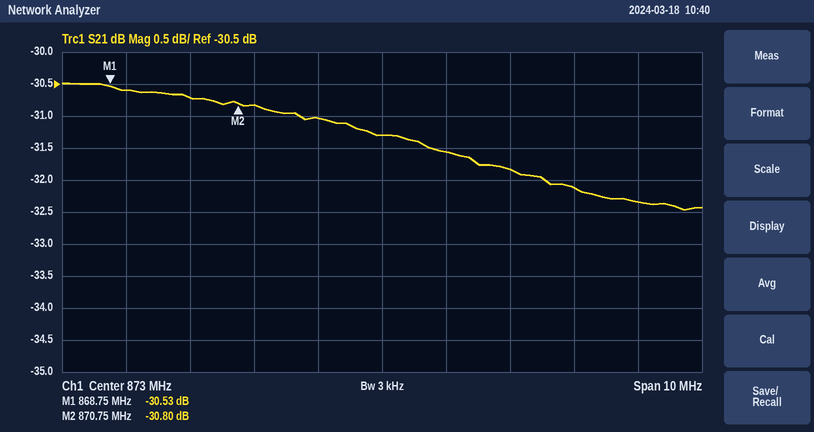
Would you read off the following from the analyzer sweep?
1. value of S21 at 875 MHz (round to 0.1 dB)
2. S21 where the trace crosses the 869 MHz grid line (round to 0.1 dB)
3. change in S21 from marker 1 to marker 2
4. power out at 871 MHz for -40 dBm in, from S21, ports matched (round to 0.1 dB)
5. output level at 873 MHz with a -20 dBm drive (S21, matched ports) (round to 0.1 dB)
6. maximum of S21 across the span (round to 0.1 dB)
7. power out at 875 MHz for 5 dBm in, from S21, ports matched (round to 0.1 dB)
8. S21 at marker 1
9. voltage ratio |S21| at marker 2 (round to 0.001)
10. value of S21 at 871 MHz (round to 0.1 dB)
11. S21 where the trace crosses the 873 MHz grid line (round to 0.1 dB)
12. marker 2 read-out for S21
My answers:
-31.8 dB
-30.6 dB
-0.27 dB
-70.8 dBm
-51.3 dBm
-30.5 dB
-26.8 dBm
-30.53 dB
0.029
-30.8 dB
-31.3 dB
-30.80 dB
